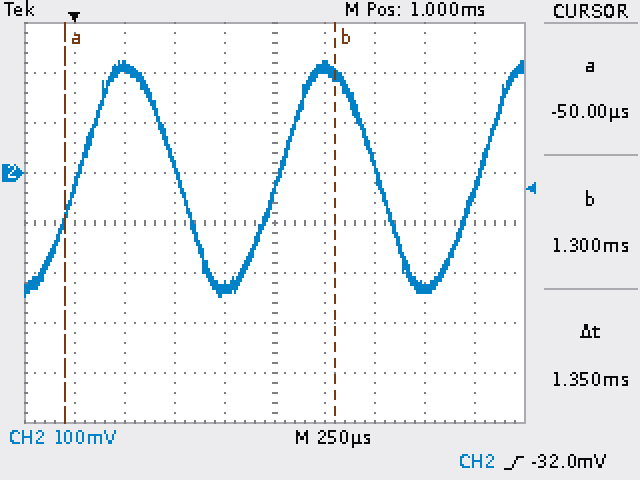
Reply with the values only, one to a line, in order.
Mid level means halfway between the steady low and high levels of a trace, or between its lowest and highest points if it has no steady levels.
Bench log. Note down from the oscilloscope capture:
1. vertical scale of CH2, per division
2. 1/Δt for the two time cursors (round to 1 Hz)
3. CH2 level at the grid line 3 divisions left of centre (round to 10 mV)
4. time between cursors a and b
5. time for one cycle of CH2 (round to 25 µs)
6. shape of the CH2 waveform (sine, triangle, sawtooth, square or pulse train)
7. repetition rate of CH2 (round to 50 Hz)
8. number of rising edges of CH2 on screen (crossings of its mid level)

100 mV
741 Hz
210 mV
1.35 ms
1.000 ms
sine
1.00 kHz
3
